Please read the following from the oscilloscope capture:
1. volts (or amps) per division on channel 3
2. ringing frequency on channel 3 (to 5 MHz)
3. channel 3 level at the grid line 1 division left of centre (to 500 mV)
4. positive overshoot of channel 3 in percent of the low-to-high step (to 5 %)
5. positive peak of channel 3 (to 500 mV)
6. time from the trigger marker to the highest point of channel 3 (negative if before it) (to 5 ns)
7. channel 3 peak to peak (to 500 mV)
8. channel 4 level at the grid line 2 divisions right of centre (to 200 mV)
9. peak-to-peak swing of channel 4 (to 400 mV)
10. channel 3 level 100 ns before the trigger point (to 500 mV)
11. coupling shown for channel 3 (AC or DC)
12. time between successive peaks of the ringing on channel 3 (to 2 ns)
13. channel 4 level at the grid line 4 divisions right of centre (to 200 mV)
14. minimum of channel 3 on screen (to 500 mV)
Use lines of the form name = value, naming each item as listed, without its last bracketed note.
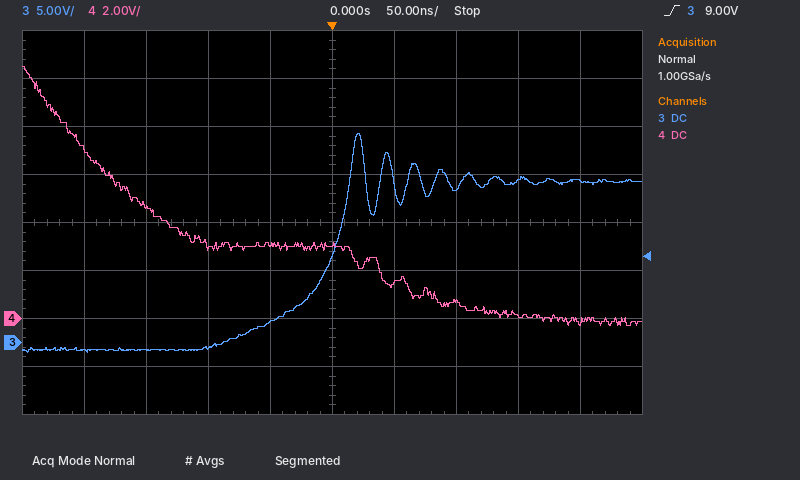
volts (or amps) per division on channel 3 = 5 V
ringing frequency on channel 3 = 45 MHz
channel 3 level at the grid line 1 division left of centre = 2.0 V
positive overshoot of channel 3 in percent of the low-to-high step = 30 %
positive peak of channel 3 = 22.0 V
time from the trigger marker to the highest point of channel 3 (negative if before it) = +20 ns
channel 3 peak to peak = 23.0 V
channel 4 level at the grid line 2 divisions right of centre = 800 mV
peak-to-peak swing of channel 4 = 10.8 V
channel 3 level 100 ns before the trigger point = -500 mV
coupling shown for channel 3 = DC
time between successive peaks of the ringing on channel 3 = 22 ns
channel 4 level at the grid line 4 divisions right of centre = -200 mV
minimum of channel 3 on screen = -1.0 V
